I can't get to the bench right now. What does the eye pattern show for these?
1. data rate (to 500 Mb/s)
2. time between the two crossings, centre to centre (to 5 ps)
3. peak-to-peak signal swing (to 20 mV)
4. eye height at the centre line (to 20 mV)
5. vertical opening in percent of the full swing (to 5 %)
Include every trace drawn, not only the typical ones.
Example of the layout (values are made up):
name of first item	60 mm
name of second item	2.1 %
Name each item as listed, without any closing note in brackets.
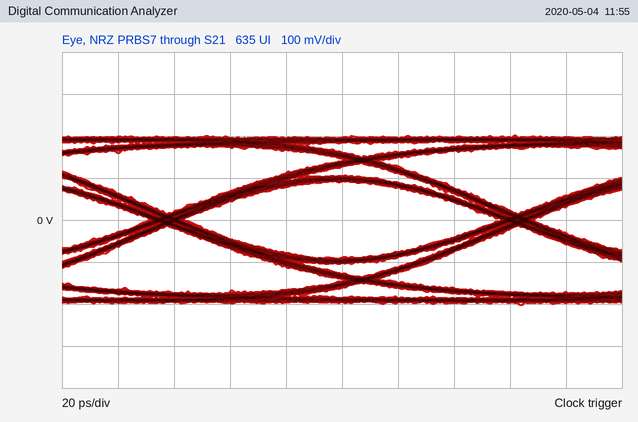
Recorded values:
data rate	8.0 Gb/s
time between the two crossings, centre to centre	125 ps
peak-to-peak signal swing	400 mV
eye height at the centre line	180 mV
vertical opening in percent of the full swing	45 %
